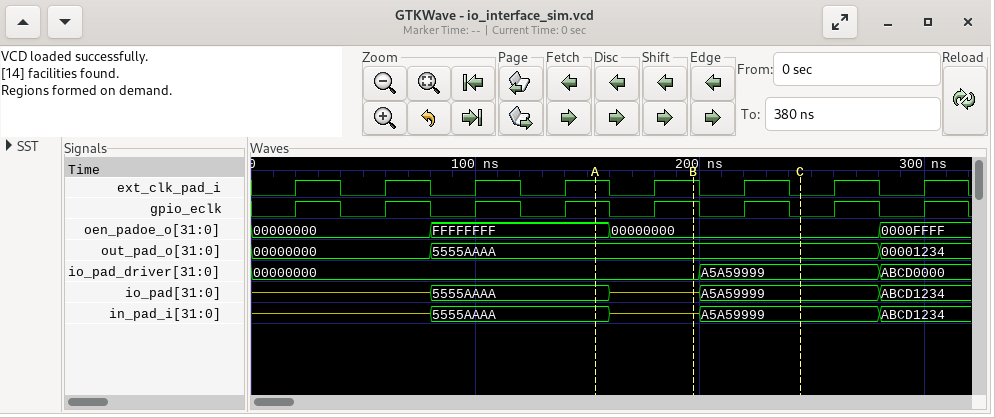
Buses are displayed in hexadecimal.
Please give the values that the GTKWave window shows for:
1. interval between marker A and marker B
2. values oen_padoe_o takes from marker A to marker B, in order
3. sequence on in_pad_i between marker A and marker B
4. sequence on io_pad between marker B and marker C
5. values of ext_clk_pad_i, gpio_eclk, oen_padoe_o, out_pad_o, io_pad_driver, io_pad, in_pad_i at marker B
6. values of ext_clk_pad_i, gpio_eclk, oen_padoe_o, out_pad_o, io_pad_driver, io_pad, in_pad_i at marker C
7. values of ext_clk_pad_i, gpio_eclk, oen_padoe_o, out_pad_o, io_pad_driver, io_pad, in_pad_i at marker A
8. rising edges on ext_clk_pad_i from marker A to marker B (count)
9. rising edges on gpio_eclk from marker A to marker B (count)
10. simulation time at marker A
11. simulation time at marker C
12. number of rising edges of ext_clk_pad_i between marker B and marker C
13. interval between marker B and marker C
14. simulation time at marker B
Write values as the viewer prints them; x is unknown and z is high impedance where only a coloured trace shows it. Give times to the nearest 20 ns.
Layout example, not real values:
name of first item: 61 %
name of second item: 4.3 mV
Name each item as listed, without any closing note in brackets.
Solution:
interval between marker A and marker B: 40 ns
values oen_padoe_o takes from marker A to marker B, in order: FFFFFFFF, 00000000
sequence on in_pad_i between marker A and marker B: 5555AAAA, z
sequence on io_pad between marker B and marker C: z, A5A59999
values of ext_clk_pad_i, gpio_eclk, oen_padoe_o, out_pad_o, io_pad_driver, io_pad, in_pad_i at marker B: ext_clk_pad_i=1, gpio_eclk=1, oen_padoe_o=00000000, out_pad_o=5555AAAA, io_pad_driver=00000000, io_pad=z, in_pad_i=z
values of ext_clk_pad_i, gpio_eclk, oen_padoe_o, out_pad_o, io_pad_driver, io_pad, in_pad_i at marker C: ext_clk_pad_i=0, gpio_eclk=0, oen_padoe_o=00000000, out_pad_o=5555AAAA, io_pad_driver=A5A59999, io_pad=A5A59999, in_pad_i=A5A59999
values of ext_clk_pad_i, gpio_eclk, oen_padoe_o, out_pad_o, io_pad_driver, io_pad, in_pad_i at marker A: ext_clk_pad_i=1, gpio_eclk=1, oen_padoe_o=FFFFFFFF, out_pad_o=5555AAAA, io_pad_driver=00000000, io_pad=5555AAAA, in_pad_i=5555AAAA
rising edges on ext_clk_pad_i from marker A to marker B: 1
rising edges on gpio_eclk from marker A to marker B: 1
simulation time at marker A: 160 ns
simulation time at marker C: 240 ns
number of rising edges of ext_clk_pad_i between marker B and marker C: 1
interval between marker B and marker C: 40 ns
simulation time at marker B: 200 ns
